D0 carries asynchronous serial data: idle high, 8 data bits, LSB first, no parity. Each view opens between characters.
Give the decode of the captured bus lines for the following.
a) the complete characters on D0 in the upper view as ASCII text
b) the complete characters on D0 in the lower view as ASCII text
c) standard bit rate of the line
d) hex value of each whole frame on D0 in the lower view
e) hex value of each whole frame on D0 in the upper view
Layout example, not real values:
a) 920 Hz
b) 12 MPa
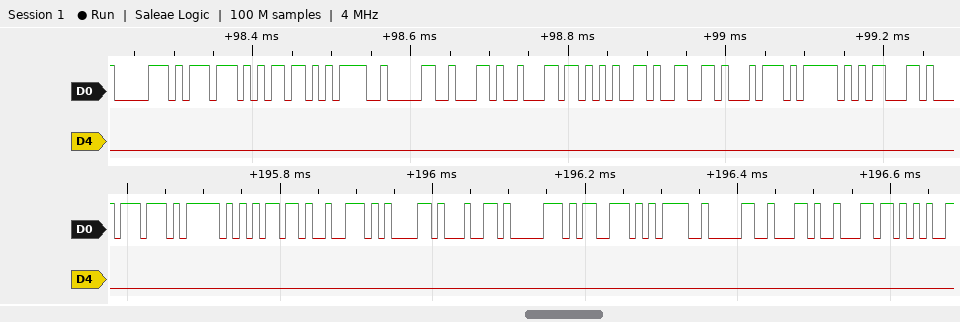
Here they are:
a) "pwm=0,left_c"
b) "w_mradps=0,l"
c) 115200 baud
d) 77, 5F, 6D, 72, 61, 64, 70, 73, 3D, 30, 2C, 6C
e) 70, 77, 6D, 3D, 30, 2C, 6C, 65, 66, 74, 5F, 63
